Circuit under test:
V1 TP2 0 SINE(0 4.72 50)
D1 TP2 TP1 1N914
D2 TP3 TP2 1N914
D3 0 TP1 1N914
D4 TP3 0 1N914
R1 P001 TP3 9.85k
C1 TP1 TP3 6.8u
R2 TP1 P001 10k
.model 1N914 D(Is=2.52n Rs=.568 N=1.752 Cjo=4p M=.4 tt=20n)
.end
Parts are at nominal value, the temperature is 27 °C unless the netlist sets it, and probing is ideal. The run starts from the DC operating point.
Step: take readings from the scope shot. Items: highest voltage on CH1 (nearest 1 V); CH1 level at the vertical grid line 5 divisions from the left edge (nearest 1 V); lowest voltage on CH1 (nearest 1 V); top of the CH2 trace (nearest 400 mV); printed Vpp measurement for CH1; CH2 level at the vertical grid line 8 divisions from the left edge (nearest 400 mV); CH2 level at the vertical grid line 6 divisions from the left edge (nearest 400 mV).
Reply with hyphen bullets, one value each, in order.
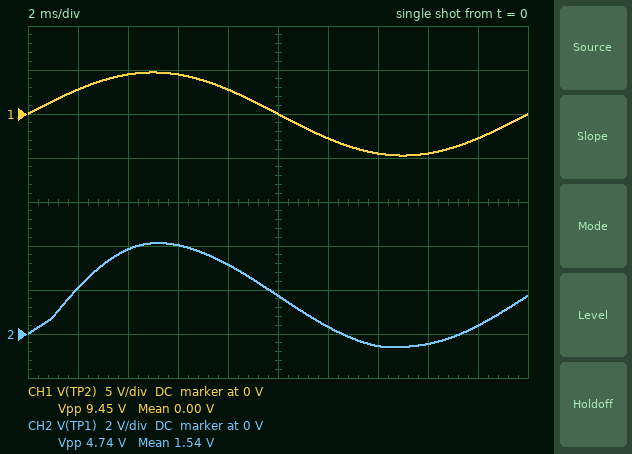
- 5 V
- 0 V
- -5 V
- 4.0 V
- 9.45 V
- -400 mV
- 400 mV
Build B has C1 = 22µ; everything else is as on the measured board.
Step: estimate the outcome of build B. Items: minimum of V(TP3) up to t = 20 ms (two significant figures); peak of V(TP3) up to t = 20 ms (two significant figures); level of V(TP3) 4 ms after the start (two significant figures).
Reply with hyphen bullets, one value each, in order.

- -4.1 V
- 750 mV
- 700 mV
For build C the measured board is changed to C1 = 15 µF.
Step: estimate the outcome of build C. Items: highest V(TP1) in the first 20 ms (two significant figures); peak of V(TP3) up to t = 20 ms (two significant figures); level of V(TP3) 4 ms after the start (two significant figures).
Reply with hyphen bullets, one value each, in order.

- 4.1 V
- 730 mV
- 680 mV
